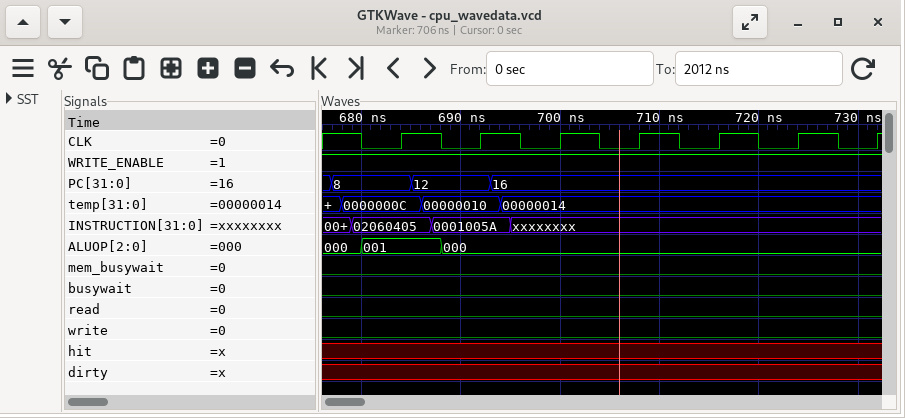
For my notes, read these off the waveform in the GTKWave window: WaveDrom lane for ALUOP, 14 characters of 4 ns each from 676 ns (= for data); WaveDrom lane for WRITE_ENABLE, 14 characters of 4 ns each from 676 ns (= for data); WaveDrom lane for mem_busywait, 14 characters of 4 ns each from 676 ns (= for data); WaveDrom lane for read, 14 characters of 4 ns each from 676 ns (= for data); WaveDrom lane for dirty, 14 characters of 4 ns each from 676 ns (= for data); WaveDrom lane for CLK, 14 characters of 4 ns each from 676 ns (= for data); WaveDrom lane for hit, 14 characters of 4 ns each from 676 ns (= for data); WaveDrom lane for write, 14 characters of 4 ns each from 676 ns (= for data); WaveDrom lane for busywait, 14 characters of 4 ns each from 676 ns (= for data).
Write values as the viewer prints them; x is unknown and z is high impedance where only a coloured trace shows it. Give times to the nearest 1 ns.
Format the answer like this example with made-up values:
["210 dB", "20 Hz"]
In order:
["{name: 'ALUOP', wave: '==.=..........', data: '000 001 000'}", "{name: 'WRITE_ENABLE', wave: '1.............'}", "{name: 'mem_busywait', wave: '0.............'}", "{name: 'read', wave: '0.............'}", "{name: 'dirty', wave: 'x.............'}", "{name: 'CLK', wave: '10101010101010'}", "{name: 'hit', wave: 'x.............'}", "{name: 'write', wave: '0.............'}", "{name: 'busywait', wave: '0.............'}"]
